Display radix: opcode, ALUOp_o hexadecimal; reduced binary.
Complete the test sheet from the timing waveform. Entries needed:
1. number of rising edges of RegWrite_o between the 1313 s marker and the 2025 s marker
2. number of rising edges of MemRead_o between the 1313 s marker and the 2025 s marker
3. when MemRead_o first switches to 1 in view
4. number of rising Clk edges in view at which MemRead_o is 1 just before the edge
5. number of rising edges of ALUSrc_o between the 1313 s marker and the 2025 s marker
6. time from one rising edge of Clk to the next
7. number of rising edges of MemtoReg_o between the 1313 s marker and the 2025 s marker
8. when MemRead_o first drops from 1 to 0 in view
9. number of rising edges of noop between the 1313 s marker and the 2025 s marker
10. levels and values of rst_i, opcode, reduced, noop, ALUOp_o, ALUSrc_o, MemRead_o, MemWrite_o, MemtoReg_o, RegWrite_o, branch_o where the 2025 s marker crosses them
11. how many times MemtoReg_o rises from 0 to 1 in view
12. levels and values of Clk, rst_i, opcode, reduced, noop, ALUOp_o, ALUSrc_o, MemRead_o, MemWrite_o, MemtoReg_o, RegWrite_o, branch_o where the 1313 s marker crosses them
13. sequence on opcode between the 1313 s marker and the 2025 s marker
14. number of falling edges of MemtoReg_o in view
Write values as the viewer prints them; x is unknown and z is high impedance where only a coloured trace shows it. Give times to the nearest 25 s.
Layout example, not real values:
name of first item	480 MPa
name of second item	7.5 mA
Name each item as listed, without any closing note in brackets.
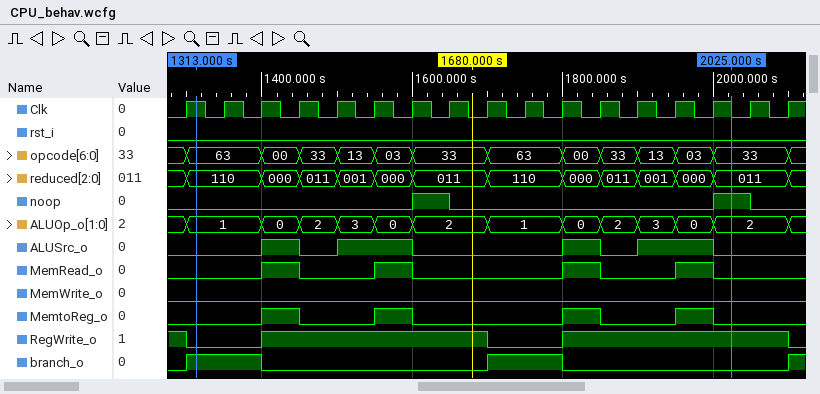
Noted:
number of rising edges of RegWrite_o between the 1313 s marker and the 2025 s marker	2
number of rising edges of MemRead_o between the 1313 s marker and the 2025 s marker	4
when MemRead_o first switches to 1 in view	1400 s
number of rising Clk edges in view at which MemRead_o is 1 just before the edge	4
number of rising edges of ALUSrc_o between the 1313 s marker and the 2025 s marker	4
time from one rising edge of Clk to the next	50 s
number of rising edges of MemtoReg_o between the 1313 s marker and the 2025 s marker	4
when MemRead_o first drops from 1 to 0 in view	1450 s
number of rising edges of noop between the 1313 s marker and the 2025 s marker	2
levels and values of rst_i, opcode, reduced, noop, ALUOp_o, ALUSrc_o, MemRead_o, MemWrite_o, MemtoReg_o, RegWrite_o, branch_o where the 2025 s marker crosses them	rst_i=0, opcode=33, reduced=011, noop=1, ALUOp_o=2, ALUSrc_o=0, MemRead_o=0, MemWrite_o=0, MemtoReg_o=0, RegWrite_o=1, branch_o=0
how many times MemtoReg_o rises from 0 to 1 in view	4
levels and values of Clk, rst_i, opcode, reduced, noop, ALUOp_o, ALUSrc_o, MemRead_o, MemWrite_o, MemtoReg_o, RegWrite_o, branch_o where the 1313 s marker crosses them	Clk=1, rst_i=0, opcode=63, reduced=110, noop=0, ALUOp_o=1, ALUSrc_o=0, MemRead_o=0, MemWrite_o=0, MemtoReg_o=0, RegWrite_o=0, branch_o=1
sequence on opcode between the 1313 s marker and the 2025 s marker	63, 00, 33, 13, 03, 33, 63, 00, 33, 13, 03, 33
number of falling edges of MemtoReg_o in view	4
